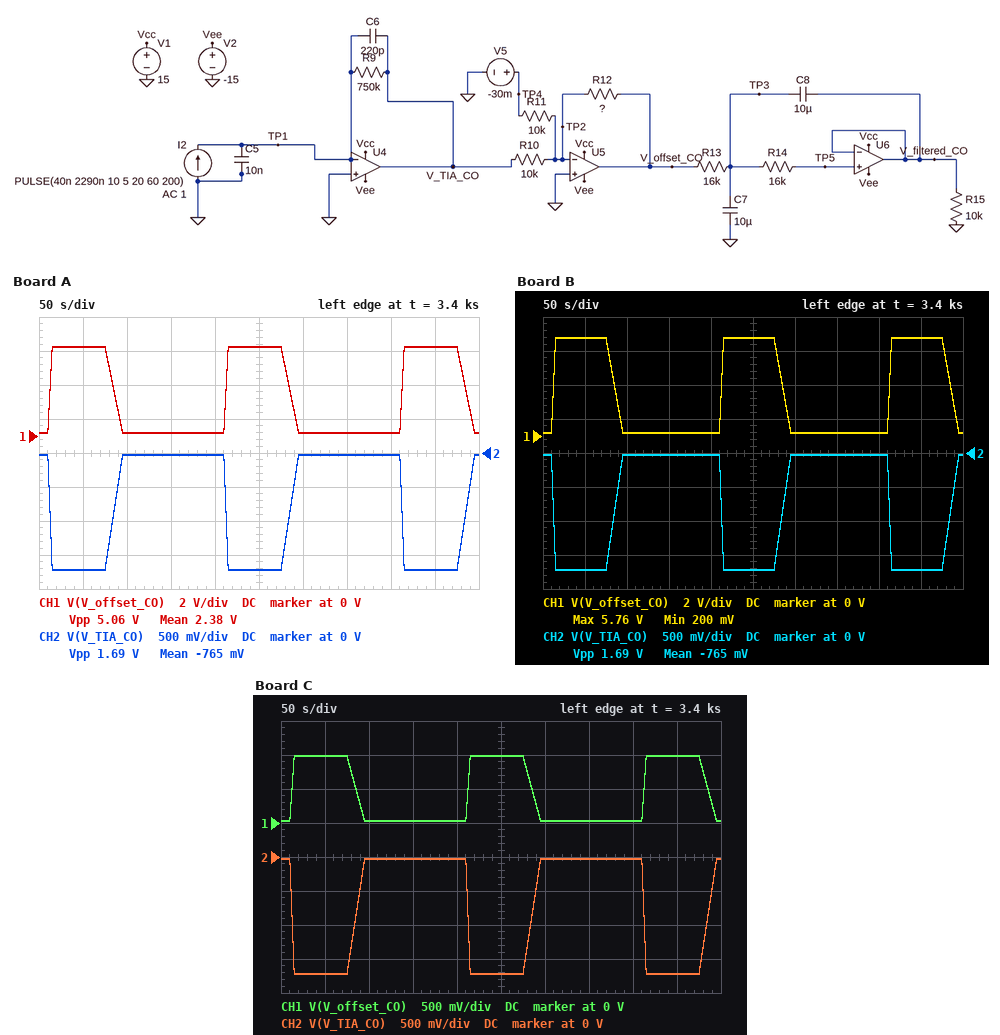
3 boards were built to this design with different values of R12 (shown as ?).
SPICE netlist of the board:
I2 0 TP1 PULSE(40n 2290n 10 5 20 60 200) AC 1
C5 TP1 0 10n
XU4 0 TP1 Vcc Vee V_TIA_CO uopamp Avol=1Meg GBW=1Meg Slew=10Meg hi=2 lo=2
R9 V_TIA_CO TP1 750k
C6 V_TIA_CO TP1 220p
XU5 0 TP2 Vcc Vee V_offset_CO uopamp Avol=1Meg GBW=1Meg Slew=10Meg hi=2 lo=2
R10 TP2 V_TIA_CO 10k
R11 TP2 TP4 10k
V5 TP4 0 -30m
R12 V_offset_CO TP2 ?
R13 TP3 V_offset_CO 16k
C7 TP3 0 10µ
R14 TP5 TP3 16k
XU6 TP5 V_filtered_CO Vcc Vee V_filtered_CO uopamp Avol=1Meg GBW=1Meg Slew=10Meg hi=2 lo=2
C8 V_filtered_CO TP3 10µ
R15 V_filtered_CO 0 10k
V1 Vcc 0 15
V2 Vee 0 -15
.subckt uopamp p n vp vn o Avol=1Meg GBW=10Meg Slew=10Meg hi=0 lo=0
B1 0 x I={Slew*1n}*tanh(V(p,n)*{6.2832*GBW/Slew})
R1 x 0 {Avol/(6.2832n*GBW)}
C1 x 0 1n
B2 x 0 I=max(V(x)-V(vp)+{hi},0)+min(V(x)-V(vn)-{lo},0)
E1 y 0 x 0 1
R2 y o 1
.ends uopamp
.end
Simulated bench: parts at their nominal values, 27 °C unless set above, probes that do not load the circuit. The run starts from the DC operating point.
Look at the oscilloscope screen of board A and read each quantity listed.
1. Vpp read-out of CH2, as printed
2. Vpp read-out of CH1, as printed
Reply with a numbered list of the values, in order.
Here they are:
1. 1.69 V
2. 5.06 V
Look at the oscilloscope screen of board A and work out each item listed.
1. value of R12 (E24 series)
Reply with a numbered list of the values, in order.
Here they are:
1. 30 kΩ
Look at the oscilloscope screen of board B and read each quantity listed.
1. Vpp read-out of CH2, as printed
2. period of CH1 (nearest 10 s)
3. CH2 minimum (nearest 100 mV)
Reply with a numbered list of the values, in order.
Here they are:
1. 1.69 V
2. 200 s
3. -1.7 V
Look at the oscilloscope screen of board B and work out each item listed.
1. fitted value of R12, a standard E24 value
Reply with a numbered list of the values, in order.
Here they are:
1. 33 kΩ
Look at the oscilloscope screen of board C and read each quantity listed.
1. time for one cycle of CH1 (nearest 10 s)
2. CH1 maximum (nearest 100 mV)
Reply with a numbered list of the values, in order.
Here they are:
1. 200 s
2. 1.0 V
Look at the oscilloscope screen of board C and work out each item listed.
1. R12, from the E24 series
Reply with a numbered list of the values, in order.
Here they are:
1. 5.6 kΩ
